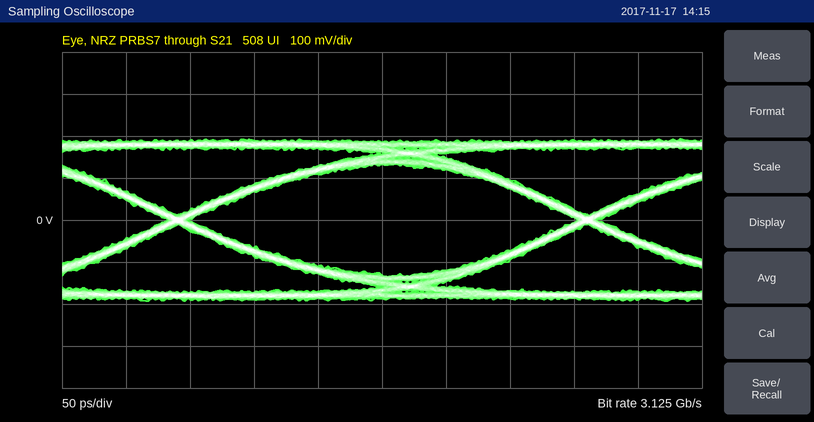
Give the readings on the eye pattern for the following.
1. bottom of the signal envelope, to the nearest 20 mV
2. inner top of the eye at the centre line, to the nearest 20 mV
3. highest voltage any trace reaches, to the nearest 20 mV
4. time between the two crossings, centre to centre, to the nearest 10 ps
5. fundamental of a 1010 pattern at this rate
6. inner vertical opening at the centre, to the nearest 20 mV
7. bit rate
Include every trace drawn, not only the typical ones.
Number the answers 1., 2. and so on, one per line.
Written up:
1. -200 mV
2. 140 mV
3. 200 mV
4. 320 ps
5. 1.5625 GHz
6. 260 mV
7. 3.125 Gb/s
